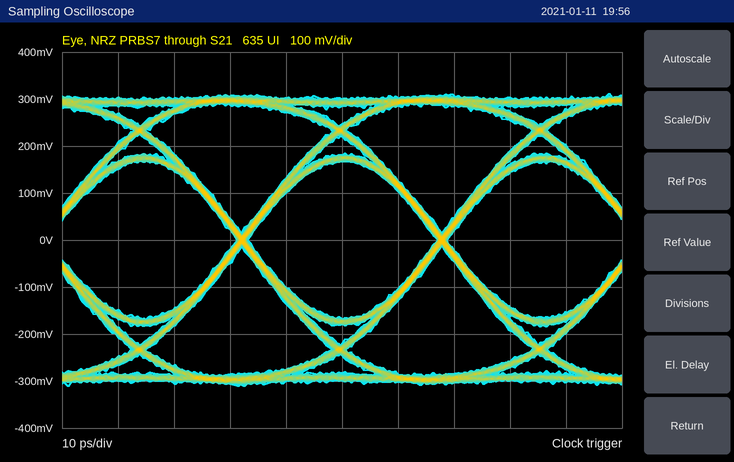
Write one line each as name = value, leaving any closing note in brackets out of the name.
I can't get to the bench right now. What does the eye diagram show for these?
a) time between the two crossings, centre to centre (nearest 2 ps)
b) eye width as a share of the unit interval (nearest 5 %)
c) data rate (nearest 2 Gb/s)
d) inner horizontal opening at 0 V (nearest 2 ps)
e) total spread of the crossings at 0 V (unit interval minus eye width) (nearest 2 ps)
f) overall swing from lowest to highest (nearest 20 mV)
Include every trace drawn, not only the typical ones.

time between the two crossings, centre to centre = 36 ps
eye width as a share of the unit interval = 95 %
data rate = 28 Gb/s
inner horizontal opening at 0 V = 34 ps
total spread of the crossings at 0 V (unit interval minus eye width) = 2 ps
overall swing from lowest to highest = 620 mV
